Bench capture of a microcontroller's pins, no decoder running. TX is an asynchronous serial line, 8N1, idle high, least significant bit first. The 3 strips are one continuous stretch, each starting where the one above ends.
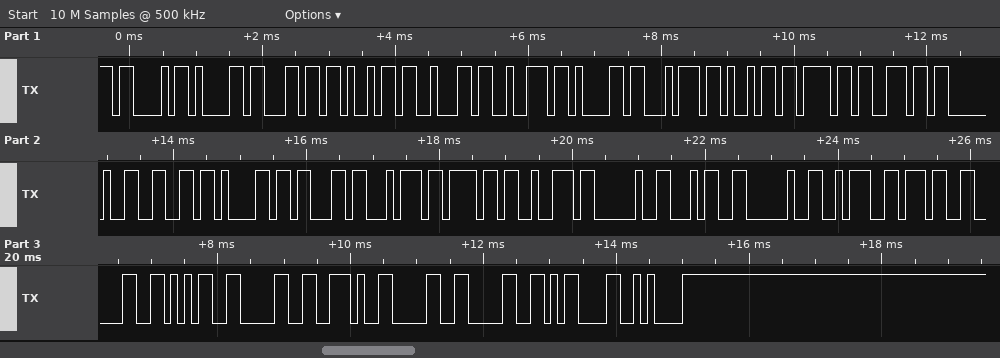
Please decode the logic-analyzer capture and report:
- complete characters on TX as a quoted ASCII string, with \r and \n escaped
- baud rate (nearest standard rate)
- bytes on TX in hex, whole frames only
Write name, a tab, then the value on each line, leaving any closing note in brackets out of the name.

complete characters on TX as a quoted ASCII string, with \r and \n escaped	"Calibration factor 4 :7050.00\r\n"
baud rate	9600 baud
bytes on TX in hex, whole frames only	0x43 0x61 0x6C 0x69 0x62 0x72 0x61 0x74 0x69 0x6F 0x6E 0x20 0x66 0x61 0x63 0x74 0x6F 0x72 0x20 0x34 0x20 0x3A 0x37 0x30 0x35 0x30 0x2E 0x30 0x30 0x0D 0x0A
